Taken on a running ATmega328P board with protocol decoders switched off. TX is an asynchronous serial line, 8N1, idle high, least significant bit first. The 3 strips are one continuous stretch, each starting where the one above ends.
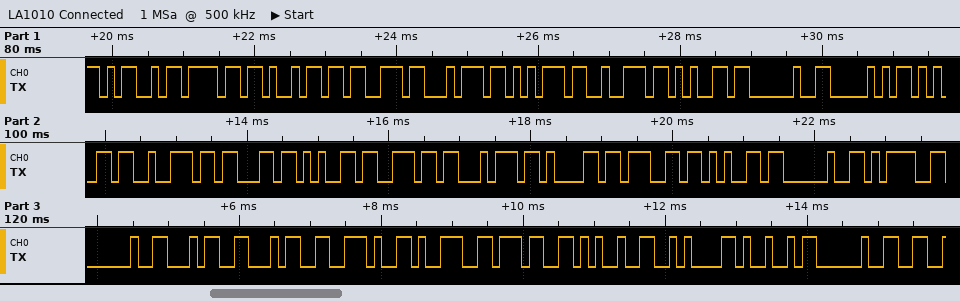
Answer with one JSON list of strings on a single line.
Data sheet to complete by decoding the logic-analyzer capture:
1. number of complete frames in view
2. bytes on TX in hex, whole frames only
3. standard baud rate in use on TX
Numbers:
["31", "4D 6F 69 73 74 75 72 65 20 50 65 72 63 65 6E 74 61 67 65 20 3D 20 34 34 2E 39 37 25 0A 49 20", "9600 baud"]
